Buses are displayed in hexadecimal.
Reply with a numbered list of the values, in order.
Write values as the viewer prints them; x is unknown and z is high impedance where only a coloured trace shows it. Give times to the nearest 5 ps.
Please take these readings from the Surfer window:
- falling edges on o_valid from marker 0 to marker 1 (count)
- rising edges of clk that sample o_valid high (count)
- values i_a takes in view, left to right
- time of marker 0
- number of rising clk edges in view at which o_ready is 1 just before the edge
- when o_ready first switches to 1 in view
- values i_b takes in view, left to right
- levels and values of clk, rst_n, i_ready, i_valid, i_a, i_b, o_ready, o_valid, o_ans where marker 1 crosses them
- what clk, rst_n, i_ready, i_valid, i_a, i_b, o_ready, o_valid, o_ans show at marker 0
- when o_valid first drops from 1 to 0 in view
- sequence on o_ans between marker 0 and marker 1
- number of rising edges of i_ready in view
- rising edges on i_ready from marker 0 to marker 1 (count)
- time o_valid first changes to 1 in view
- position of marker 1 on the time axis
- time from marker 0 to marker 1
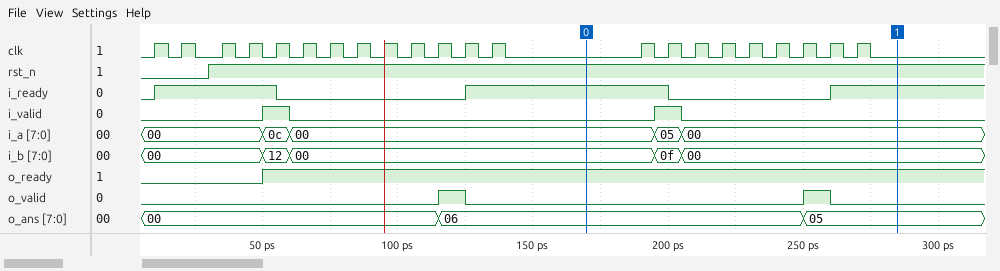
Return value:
1. 1
2. 2
3. 00, 0c, 00, 05, 00
4. 170 ps
5. 18
6. 50 ps
7. 00, 12, 00, 0f, 00
8. clk=0, rst_n=1, i_ready=1, i_valid=0, i_a=00, i_b=00, o_ready=1, o_valid=0, o_ans=05
9. clk=0, rst_n=1, i_ready=1, i_valid=0, i_a=00, i_b=00, o_ready=1, o_valid=0, o_ans=06
10. 125 ps
11. 06, 05
12. 3
13. 1
14. 115 ps
15. 285 ps
16. 115 ps
